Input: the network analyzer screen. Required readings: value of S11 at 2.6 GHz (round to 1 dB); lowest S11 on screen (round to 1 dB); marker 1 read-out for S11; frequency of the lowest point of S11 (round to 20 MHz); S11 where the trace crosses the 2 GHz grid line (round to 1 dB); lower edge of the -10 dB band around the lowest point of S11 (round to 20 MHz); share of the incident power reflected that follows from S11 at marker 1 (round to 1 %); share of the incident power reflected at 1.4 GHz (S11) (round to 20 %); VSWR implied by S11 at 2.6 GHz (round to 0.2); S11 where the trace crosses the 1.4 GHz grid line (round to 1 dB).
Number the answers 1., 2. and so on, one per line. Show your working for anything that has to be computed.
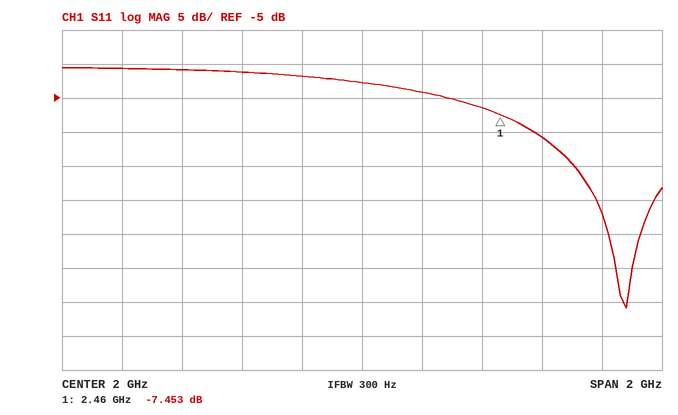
1. -11 dB
2. -36 dB
3. -7.453 dB
4. 2.88 GHz
5. -3 dB
6. 2.58 GHz
7. 10^(-7.453/10) ≈ 18 %
8. 10^(-1/10) ≈ 79.4 %, so 80 % to the nearest 20 %
9. |Γ| = 10^(-11/20) = 0.2818; VSWR = (1 + 0.2818)/(1 − 0.2818) ≈ 1.8
10. -1 dB
